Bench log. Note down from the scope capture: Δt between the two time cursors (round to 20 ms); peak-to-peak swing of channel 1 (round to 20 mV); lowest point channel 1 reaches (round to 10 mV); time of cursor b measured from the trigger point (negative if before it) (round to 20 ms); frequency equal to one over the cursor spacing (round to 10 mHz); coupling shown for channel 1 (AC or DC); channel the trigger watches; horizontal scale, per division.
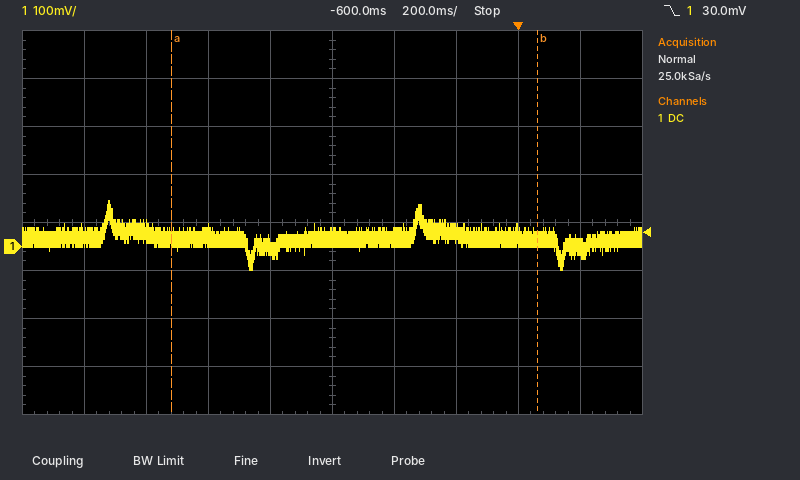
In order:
1.18 s
140 mV
-50 mV
+60 ms
850 mHz
DC
channel 1
200 ms
